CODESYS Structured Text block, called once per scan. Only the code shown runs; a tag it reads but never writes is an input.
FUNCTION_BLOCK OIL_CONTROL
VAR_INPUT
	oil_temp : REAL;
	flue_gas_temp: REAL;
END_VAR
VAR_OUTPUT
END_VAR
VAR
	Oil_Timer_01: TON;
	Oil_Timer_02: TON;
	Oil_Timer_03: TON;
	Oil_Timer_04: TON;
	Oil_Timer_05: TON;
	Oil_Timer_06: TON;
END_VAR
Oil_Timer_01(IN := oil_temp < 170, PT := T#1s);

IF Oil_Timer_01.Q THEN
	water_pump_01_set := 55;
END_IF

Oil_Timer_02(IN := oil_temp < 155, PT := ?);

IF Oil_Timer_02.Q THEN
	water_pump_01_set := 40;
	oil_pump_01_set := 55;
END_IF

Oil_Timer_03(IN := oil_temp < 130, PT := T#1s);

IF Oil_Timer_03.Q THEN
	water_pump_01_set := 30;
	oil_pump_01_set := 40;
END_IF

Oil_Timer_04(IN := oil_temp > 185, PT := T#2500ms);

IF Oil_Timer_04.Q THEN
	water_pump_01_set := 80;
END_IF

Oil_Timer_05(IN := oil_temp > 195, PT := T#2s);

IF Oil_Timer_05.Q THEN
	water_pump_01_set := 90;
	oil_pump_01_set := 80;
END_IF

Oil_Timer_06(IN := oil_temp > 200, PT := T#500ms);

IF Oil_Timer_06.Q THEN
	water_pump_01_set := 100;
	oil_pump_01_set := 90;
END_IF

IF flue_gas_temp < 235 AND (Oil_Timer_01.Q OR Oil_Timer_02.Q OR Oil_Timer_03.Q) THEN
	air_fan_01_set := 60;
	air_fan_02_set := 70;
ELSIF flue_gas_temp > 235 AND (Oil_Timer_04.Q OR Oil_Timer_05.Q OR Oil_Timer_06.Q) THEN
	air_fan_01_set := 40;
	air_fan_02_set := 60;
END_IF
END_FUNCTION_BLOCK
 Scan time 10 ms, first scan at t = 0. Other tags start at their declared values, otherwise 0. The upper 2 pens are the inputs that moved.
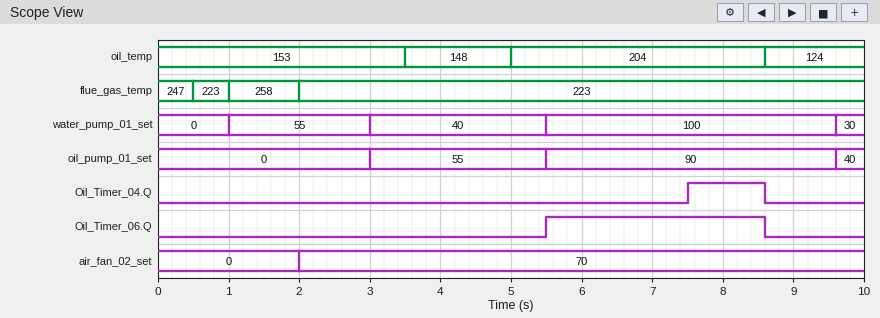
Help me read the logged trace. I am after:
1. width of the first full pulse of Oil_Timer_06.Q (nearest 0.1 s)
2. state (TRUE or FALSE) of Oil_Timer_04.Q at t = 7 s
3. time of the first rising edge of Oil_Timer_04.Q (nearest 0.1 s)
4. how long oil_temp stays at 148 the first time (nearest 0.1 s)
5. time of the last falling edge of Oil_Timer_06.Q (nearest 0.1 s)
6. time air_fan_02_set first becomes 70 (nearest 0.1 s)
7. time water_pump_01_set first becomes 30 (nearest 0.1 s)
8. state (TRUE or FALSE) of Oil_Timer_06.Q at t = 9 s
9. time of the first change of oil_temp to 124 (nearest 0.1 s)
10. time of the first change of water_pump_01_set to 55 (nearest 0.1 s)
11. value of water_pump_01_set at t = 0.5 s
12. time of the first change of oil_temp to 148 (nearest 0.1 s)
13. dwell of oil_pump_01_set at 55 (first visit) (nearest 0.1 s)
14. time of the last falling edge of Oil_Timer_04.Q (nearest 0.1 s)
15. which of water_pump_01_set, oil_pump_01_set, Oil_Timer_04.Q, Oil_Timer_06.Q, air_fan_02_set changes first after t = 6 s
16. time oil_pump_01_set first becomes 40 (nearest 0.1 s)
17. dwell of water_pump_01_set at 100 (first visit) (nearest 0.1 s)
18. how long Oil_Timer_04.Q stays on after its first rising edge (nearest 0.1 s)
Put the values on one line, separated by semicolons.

3.1 s; FALSE; 7.5 s; 1.5 s; 8.6 s; 2.0 s; 9.6 s; FALSE; 8.6 s; 1.0 s; 0; 3.5 s; 2.5 s; 8.6 s; Oil_Timer_04.Q; 9.6 s; 4.1 s; 1.1 s
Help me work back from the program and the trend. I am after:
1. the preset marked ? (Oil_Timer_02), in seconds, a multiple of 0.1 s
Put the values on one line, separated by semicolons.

3.0 s
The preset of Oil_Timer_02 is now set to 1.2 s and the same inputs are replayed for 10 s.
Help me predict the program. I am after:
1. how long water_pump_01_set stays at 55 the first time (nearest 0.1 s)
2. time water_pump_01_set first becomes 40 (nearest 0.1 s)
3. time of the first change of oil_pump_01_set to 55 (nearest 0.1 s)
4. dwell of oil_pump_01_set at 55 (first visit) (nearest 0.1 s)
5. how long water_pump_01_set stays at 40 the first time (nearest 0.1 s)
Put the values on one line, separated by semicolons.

0.2 s; 1.2 s; 1.2 s; 4.3 s; 4.3 s
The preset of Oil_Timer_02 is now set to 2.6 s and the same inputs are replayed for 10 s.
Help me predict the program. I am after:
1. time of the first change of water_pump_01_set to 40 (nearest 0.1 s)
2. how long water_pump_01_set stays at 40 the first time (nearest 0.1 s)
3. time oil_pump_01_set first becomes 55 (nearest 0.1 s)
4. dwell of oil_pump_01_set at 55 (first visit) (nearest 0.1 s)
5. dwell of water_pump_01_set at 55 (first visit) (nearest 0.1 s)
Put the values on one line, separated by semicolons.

2.6 s; 2.9 s; 2.6 s; 2.9 s; 1.6 s
